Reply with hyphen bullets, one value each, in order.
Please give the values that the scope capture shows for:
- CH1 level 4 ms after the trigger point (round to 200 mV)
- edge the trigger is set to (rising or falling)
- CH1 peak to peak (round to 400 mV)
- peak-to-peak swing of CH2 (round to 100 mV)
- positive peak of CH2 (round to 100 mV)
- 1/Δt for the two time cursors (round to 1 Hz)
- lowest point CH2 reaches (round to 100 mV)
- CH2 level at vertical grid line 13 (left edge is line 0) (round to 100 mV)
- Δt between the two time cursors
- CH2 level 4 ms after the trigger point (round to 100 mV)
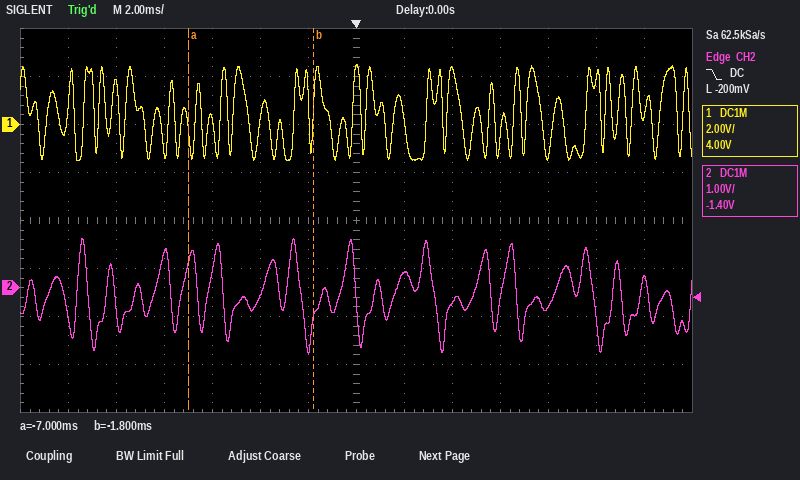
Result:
- 2.2 V
- falling
- 4.0 V
- 2.4 V
- 1.0 V
- 192 Hz
- -1.4 V
- 200 mV
- 5.2 ms
- -300 mV
